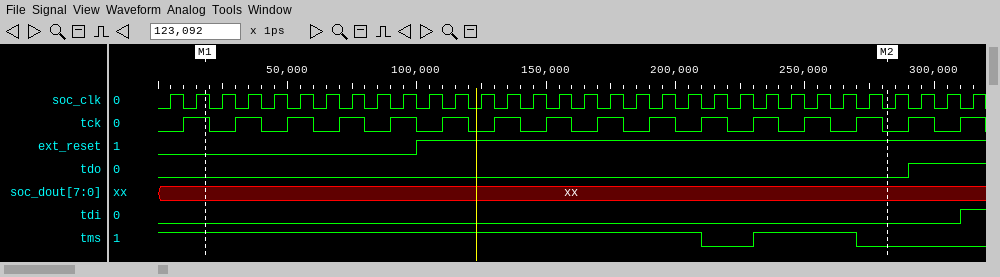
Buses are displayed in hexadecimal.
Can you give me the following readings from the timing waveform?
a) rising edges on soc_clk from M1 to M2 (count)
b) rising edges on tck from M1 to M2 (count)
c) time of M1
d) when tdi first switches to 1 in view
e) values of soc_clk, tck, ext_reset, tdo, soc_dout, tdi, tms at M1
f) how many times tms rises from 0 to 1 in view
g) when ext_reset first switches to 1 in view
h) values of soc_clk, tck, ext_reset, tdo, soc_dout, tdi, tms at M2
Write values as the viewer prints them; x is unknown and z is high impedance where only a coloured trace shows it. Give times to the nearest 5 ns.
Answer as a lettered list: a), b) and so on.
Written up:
a) 26
b) 13
c) 20 ns
d) 310 ns
e) soc_clk=1, tck=1, ext_reset=0, tdo=0, soc_dout=xx, tdi=0, tms=1
f) 1
g) 100 ns
h) soc_clk=0, tck=0, ext_reset=1, tdo=0, soc_dout=xx, tdi=0, tms=0
